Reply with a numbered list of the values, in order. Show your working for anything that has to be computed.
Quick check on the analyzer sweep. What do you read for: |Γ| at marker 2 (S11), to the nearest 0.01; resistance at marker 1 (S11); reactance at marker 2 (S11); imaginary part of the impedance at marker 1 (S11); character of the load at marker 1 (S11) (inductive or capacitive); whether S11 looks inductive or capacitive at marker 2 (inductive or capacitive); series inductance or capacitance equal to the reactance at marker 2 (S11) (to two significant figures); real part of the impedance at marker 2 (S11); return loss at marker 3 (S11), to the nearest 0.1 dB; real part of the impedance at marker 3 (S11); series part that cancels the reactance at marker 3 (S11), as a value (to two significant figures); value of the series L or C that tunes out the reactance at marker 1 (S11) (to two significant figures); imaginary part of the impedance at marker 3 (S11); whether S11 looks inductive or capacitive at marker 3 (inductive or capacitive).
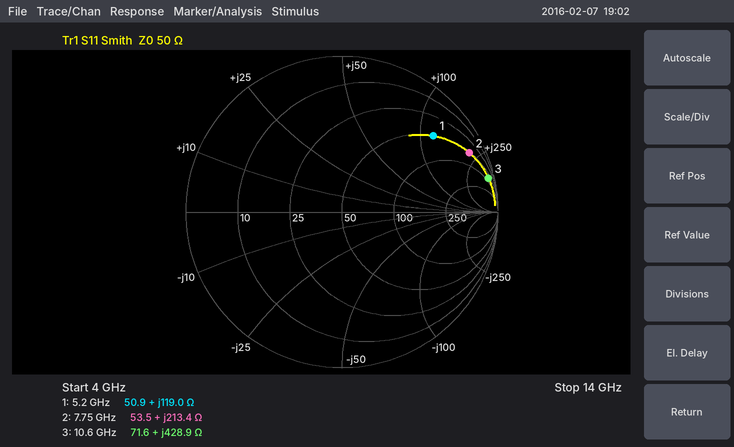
1. 0.90
2. 50.9 Ω
3. +213.4 Ω
4. +119.0 Ω
5. inductive
6. inductive
7. L = 213.4 Ω/(2π × 7.75 GHz) ≈ 4.4 nH
8. 53.5 Ω
9. 0.3 dB
10. 71.6 Ω
11. C = 1/(2π × 10.6 GHz × 428.9 Ω) ≈ 35 fF
12. C = 1/(2π × 5.2 GHz × 119 Ω) ≈ 257 fF, so 260 fF to two significant figures
13. +428.9 Ω
14. inductive
